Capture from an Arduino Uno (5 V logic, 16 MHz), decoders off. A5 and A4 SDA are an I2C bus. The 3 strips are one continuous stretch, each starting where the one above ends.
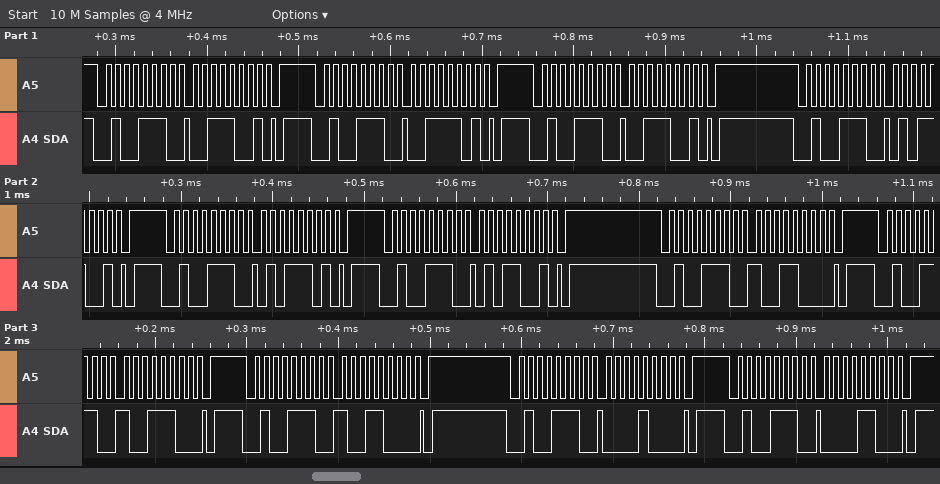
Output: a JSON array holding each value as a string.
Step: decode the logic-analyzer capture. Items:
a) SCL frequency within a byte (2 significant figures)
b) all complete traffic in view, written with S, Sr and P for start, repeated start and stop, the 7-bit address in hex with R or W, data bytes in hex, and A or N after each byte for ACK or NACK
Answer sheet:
["100 kHz", "S 27W A 39 A P S 27W A 3D A P S 27W A 39 A P S 27W A 59 A P S 27W A 5D A P S 27W A 59 A P S 27W A 98 A P S 27W A 9C A P S 27W A 98 A P S 27W A 08 A P S 27W A 0C A P"]
